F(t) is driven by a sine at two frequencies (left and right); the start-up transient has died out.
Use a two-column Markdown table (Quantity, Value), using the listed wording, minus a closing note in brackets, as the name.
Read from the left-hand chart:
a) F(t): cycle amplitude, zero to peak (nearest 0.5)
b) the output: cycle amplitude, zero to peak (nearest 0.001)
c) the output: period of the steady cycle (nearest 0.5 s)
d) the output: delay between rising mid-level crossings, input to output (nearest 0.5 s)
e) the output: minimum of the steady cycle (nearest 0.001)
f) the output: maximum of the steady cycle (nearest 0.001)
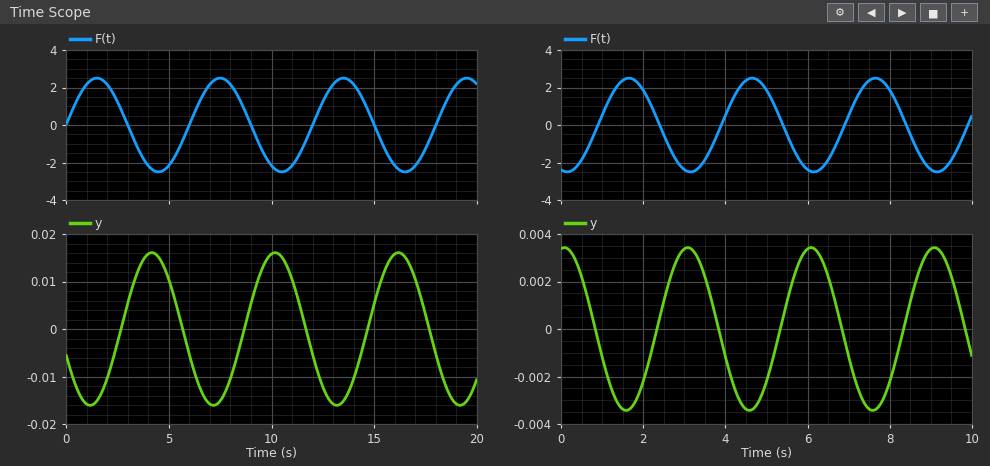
| Quantity | Value |
|---|---|
| F(t): cycle amplitude, zero to peak | 2.5 |
| the output: cycle amplitude, zero to peak | 0.016 |
| the output: period of the steady cycle | 6.0 s |
| the output: delay between rising mid-level crossings, input to output | 2.5 s |
| the output: minimum of the steady cycle | -0.016 |
| the output: maximum of the steady cycle | 0.016 |
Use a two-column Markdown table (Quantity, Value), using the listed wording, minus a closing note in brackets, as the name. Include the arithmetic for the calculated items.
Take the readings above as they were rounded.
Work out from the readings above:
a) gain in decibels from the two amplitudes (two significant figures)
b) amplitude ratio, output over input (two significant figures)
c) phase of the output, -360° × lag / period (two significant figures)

| Quantity | Value |
|---|---|
| gain in decibels from the two amplitudes | 20 log10(0.016 / 2.5) = -44 dB |
| amplitude ratio, output over input | 0.016 / 2.5 = 0.0064 |
| phase of the output, -360° × lag / period | -360 × 2.5 / 6 = -150° |
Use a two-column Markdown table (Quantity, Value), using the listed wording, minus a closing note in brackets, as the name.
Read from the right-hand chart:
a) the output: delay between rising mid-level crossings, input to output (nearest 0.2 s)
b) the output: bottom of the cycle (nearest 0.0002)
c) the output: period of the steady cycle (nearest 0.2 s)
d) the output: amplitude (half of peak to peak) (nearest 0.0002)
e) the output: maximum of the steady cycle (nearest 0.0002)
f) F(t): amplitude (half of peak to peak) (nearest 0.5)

| Quantity | Value |
|---|---|
| the output: delay between rising mid-level crossings, input to output | 1.4 s |
| the output: bottom of the cycle | -0.0034 |
| the output: period of the steady cycle | 3.0 s |
| the output: amplitude (half of peak to peak) | 0.0034 |
| the output: maximum of the steady cycle | 0.0034 |
| F(t): amplitude (half of peak to peak) | 2.5 |
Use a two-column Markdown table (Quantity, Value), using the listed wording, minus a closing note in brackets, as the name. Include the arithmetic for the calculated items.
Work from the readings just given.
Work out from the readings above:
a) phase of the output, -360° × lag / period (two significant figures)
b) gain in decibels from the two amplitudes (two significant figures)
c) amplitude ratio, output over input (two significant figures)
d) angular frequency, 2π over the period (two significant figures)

| Quantity | Value |
|---|---|
| phase of the output, -360° × lag / period | -360 × 1.4 / 3 = -170° |
| gain in decibels from the two amplitudes | 20 log10(0.0034 / 2.5) = -57 dB |
| amplitude ratio, output over input | 0.0034 / 2.5 = 0.0014 |
| angular frequency, 2π over the period | 2π / 3 = 2.1 rad/s |
